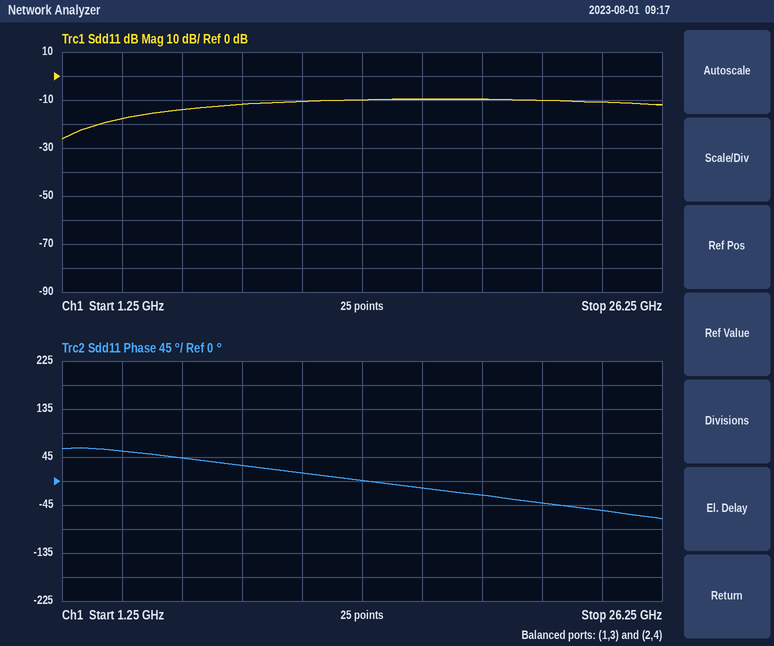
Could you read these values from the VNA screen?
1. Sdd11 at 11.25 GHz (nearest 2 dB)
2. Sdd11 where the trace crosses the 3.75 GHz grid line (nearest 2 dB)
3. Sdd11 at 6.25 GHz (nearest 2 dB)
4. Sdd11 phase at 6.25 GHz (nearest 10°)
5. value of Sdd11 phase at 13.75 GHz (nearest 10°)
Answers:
-10 dB
-18 dB
-14 dB
40°
0°
